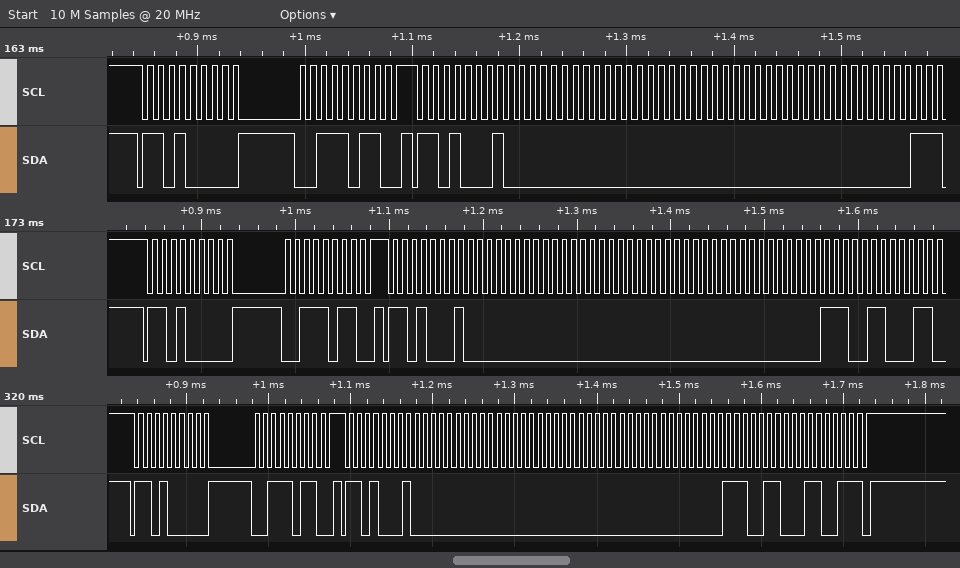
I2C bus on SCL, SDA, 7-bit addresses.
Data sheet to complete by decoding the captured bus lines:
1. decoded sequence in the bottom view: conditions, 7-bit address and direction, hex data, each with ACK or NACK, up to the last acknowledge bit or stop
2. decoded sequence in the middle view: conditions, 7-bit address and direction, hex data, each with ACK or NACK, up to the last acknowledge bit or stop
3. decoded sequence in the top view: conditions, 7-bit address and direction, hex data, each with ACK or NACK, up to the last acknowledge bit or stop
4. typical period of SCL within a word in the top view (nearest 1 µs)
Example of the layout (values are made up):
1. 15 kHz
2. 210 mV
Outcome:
1. start, address 68 write ACK, 3B ACK, stop, start, address 68 read ACK, 00 ACK, 00 ACK, 00 ACK, 00 ACK, 73 ACK, 33 NACK, stop
2. start, address 68 write ACK, 3B ACK, stop, start, address 68 read ACK, 00 ACK, 00 ACK, 00 ACK, 00 ACK, 73 ACK
3. start, address 68 write ACK, 3B ACK, stop, start, address 68 read ACK, 00 ACK, 00 ACK, 00 ACK, 00 ACK
4. 10 µs
